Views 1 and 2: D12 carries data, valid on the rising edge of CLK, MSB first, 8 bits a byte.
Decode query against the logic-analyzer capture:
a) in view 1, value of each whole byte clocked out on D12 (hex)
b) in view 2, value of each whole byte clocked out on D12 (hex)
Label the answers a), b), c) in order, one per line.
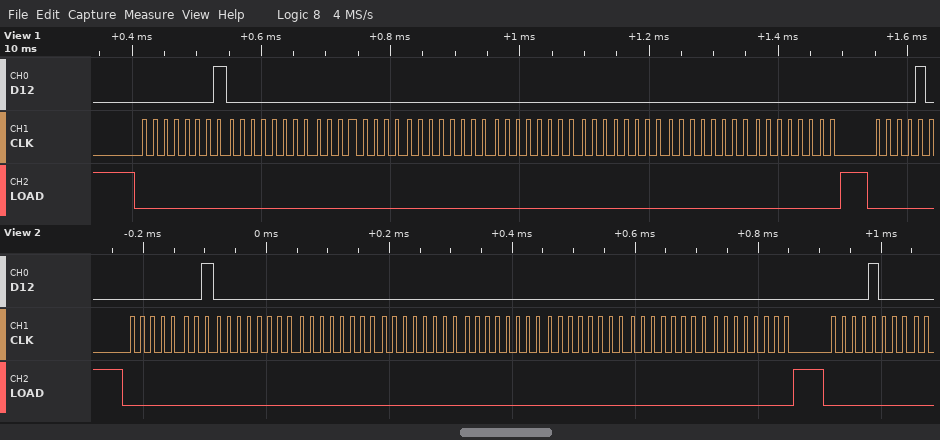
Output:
a) 0x01 0x00 0x00 0x00 0x00 0x00 0x00 0x00
b) 0x01 0x00 0x00 0x00 0x00 0x00 0x00 0x00 0x08
